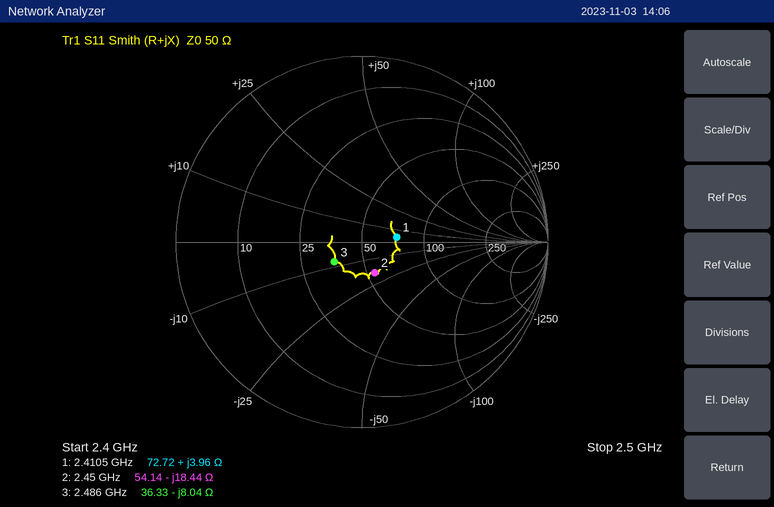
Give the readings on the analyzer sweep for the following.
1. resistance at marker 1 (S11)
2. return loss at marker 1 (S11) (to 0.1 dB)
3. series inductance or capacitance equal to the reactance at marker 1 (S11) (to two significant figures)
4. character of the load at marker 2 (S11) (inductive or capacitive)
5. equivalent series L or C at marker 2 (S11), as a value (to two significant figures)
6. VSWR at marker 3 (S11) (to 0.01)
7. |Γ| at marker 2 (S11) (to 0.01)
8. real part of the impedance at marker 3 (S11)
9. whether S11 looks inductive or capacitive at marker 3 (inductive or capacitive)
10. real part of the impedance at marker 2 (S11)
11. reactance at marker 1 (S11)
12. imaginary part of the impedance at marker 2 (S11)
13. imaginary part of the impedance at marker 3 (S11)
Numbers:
72.72 Ω
14.5 dB
260 pH
capacitive
3.5 pF
1.45
0.18
36.33 Ω
capacitive
54.14 Ω
+3.96 Ω
-18.44 Ω
-8.04 Ω
